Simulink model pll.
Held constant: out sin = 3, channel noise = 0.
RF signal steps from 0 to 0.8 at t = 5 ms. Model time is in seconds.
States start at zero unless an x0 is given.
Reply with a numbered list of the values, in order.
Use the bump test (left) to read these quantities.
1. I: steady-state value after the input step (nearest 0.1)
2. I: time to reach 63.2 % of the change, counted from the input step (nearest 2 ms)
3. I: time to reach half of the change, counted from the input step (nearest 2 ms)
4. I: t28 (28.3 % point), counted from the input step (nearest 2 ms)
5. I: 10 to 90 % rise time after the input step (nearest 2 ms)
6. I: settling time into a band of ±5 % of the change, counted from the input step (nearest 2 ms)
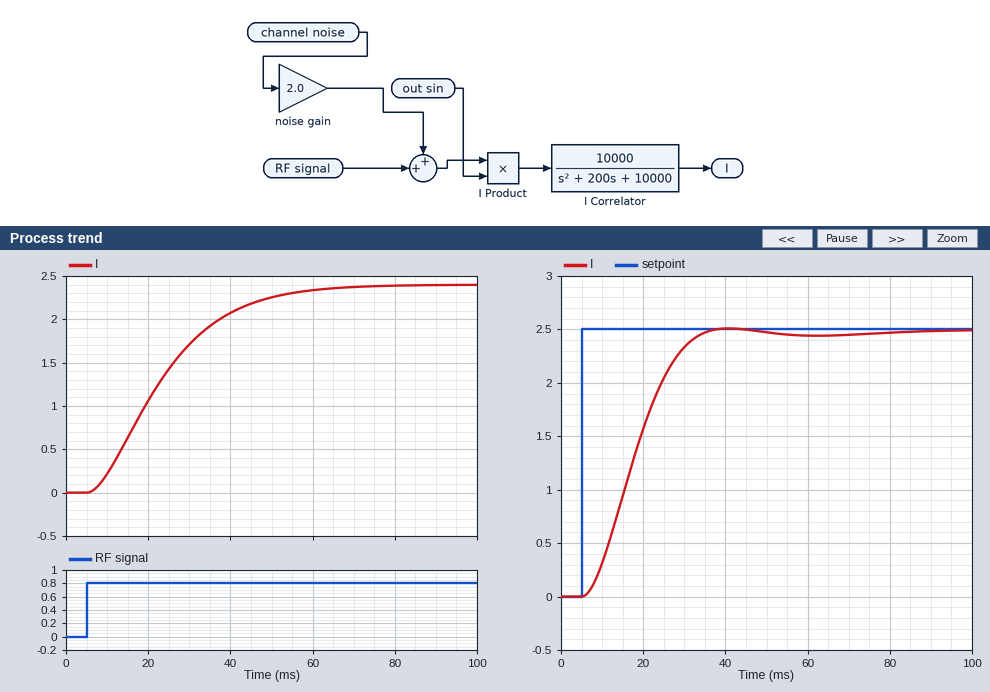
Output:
1. 2.4
2. 22 ms
3. 16 ms
4. 10 ms
5. 34 ms
6. 48 ms
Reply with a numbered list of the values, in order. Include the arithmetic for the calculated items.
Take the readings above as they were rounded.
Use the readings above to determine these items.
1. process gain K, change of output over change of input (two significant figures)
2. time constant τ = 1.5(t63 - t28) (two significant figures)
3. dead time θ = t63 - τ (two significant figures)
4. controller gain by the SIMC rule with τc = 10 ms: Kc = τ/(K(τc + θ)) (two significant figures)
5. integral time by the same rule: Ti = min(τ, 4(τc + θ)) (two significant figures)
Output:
1. (2.4 - 0) / 0.8 = 3.0
2. 1.5 × (22 - 10) = 18 ms
3. 22 - 18 = 4.0 ms
4. 18 / (3 × (10 + 4)) = 0.43
5. min(18, 4 × (10 + 4)) = 18 ms
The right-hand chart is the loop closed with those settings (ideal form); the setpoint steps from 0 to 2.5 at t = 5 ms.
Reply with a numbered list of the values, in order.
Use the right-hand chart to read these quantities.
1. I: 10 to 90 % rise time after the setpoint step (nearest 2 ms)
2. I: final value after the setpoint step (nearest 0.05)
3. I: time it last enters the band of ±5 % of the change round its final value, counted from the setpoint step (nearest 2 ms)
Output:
1. 18 ms
2. 2.50
3. 26 ms
